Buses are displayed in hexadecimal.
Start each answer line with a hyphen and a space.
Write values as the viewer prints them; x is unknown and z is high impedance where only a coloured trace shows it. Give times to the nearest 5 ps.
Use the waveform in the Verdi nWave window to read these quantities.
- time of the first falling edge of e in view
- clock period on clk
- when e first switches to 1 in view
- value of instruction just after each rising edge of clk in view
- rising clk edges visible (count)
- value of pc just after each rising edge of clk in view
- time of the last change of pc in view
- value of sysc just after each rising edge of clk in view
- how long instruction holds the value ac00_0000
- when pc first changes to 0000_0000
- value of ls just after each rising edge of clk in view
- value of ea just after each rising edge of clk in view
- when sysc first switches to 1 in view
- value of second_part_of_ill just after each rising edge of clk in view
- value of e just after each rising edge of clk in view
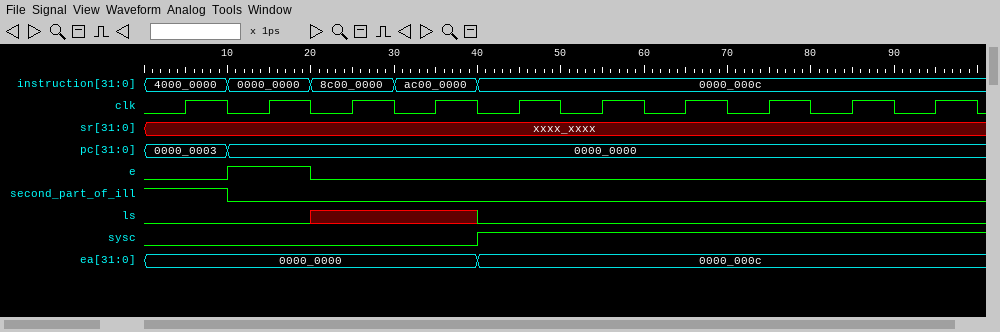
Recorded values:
- 20 ps
- 10 ps
- 10 ps
- 4000_0000, 0000_0000, 8c00_0000, ac00_0000, 0000_000c, 0000_000c, 0000_000c, 0000_000c, 0000_000c, 0000_000c
- 10
- 0000_0003, 0000_0000, 0000_0000, 0000_0000, 0000_0000, 0000_0000, 0000_0000, 0000_0000, 0000_0000, 0000_0000
- 10 ps
- 0 0 0 0 1 1 1 1 1 1
- 10 ps
- 10 ps
- 0 0 x x 0 0 0 0 0 0
- 0000_0000, 0000_0000, 0000_0000, 0000_0000, 0000_000c, 0000_000c, 0000_000c, 0000_000c, 0000_000c, 0000_000c
- 40 ps
- 1 0 0 0 0 0 0 0 0 0
- 0 1 0 0 0 0 0 0 0 0
